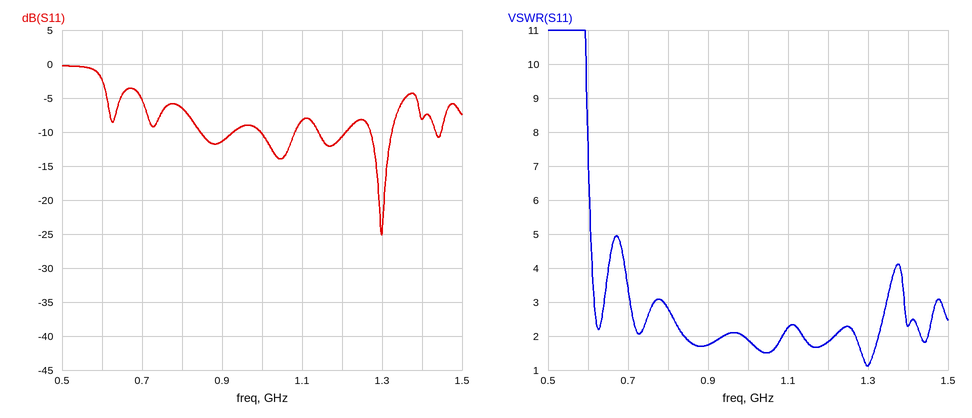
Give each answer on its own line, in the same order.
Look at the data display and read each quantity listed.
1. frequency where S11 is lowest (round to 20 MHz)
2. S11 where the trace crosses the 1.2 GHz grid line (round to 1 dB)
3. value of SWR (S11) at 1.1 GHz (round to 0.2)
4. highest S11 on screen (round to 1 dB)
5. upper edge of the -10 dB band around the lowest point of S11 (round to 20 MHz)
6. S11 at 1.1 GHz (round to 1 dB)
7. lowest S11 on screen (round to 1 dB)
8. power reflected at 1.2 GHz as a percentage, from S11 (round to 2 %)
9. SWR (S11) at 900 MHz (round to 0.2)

1.30 GHz
-11 dB
2.2
0 dB
1.32 GHz
-8 dB
-25 dB
8 %
1.8
